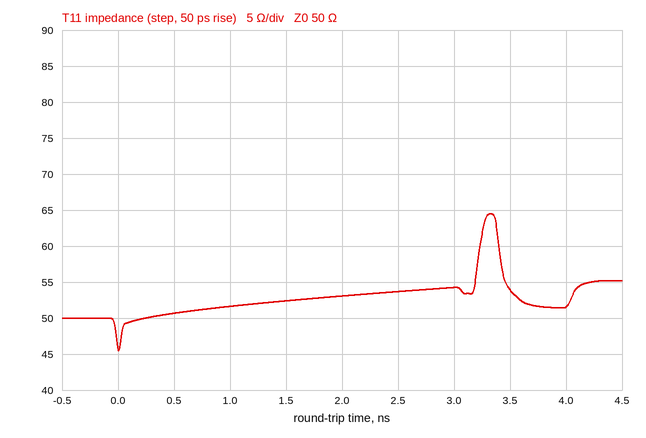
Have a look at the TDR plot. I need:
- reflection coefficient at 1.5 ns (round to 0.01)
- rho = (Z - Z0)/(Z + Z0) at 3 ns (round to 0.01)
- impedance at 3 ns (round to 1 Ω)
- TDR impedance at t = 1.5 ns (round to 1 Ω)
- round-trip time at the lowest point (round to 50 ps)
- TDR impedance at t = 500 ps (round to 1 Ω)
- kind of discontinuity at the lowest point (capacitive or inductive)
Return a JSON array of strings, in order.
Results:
["+0.02", "+0.04", "54 Ω", "52 Ω", "0 ps", "51 Ω", "capacitive"]
